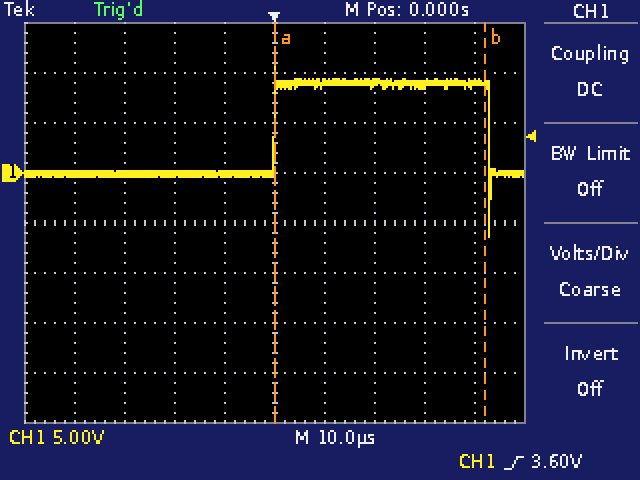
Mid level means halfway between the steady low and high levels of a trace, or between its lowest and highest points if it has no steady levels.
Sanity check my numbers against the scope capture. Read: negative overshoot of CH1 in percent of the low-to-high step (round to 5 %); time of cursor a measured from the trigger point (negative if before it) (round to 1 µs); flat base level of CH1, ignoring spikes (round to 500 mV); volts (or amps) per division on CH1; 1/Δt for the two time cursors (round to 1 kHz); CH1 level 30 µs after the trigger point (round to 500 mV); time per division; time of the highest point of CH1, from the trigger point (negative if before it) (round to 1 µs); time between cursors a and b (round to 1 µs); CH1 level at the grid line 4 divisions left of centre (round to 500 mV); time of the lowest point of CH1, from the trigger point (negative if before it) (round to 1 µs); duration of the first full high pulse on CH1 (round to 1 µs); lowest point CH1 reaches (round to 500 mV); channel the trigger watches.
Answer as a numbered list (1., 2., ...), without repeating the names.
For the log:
1. 70 %
2. 0 µs
3. 0.0 V
4. 5 V
5. 24 kHz
6. 9.0 V
7. 10 µs
8. 0 µs
9. 42 µs
10. 0.0 V
11. +43 µs
12. 43 µs
13. -6.5 V
14. CH1
